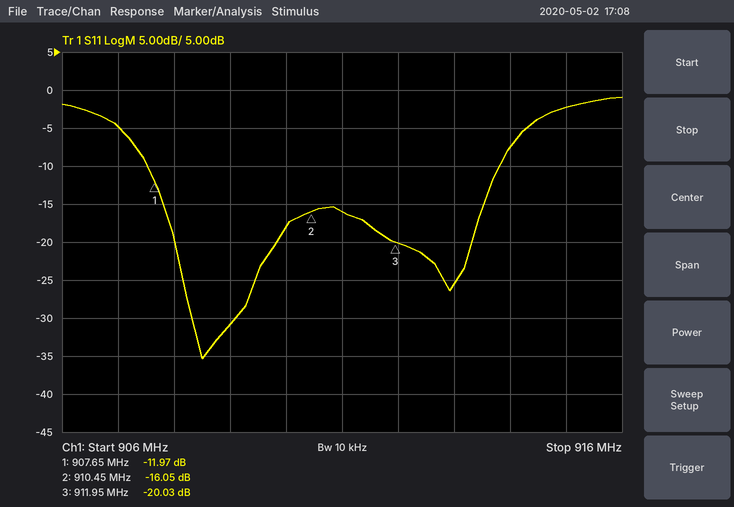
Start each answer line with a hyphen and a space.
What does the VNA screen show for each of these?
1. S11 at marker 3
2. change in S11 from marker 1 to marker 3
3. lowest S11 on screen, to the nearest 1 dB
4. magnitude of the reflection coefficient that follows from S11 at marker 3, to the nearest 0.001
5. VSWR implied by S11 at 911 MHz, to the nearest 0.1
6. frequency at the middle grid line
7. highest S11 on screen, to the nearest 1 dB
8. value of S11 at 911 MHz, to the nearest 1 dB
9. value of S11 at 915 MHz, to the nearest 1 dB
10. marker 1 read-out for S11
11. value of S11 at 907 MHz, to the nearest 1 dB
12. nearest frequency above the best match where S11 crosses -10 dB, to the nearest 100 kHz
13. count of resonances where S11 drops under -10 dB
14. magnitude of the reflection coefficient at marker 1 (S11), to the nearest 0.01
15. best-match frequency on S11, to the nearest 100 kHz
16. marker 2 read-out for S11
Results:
- -20.03 dB
- -8.06 dB
- -35 dB
- 0.100
- 1.4
- 911 MHz
- -1 dB
- -16 dB
- -2 dB
- -11.97 dB
- -5 dB
- 913.8 MHz
- 2
- 0.25
- 908.5 MHz
- -16.05 dB
